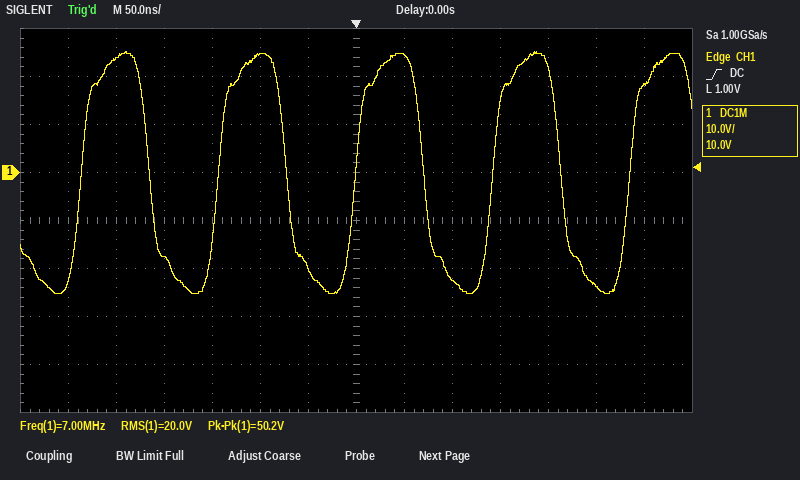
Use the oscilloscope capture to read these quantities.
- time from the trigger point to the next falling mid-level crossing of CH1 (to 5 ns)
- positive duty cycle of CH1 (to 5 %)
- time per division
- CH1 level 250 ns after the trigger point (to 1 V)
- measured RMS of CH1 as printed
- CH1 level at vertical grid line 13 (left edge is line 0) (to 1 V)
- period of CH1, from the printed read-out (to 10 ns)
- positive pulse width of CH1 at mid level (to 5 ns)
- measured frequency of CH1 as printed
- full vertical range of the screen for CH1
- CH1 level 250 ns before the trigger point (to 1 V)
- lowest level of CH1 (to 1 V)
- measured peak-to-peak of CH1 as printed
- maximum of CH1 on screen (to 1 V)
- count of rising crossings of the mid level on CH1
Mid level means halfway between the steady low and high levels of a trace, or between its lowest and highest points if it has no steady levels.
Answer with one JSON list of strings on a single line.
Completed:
["70 ns", "50 %", "50 ns", "-24 V", "20.0 V", "18 V", "140 ns", "70 ns", "7.00 MHz", "80 V", "24 V", "-25 V", "50.2 V", "25 V", "5"]
